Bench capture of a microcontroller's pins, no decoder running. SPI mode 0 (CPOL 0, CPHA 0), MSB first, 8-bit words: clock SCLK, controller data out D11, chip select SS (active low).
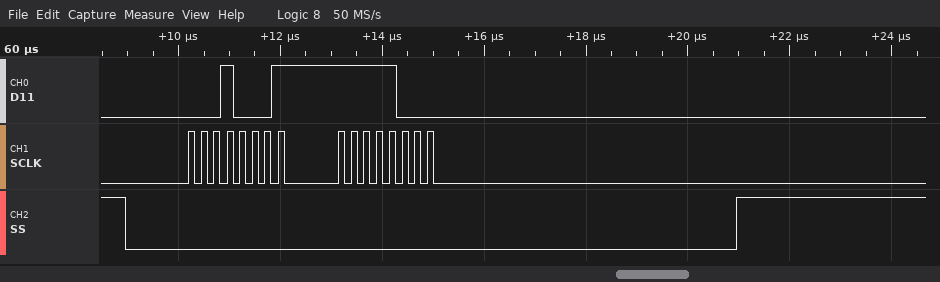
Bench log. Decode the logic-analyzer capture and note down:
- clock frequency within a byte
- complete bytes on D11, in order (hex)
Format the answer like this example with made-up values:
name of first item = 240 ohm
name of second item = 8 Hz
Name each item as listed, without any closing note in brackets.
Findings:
clock frequency within a byte = 4 MHz
complete bytes on D11, in order = 11 F8
